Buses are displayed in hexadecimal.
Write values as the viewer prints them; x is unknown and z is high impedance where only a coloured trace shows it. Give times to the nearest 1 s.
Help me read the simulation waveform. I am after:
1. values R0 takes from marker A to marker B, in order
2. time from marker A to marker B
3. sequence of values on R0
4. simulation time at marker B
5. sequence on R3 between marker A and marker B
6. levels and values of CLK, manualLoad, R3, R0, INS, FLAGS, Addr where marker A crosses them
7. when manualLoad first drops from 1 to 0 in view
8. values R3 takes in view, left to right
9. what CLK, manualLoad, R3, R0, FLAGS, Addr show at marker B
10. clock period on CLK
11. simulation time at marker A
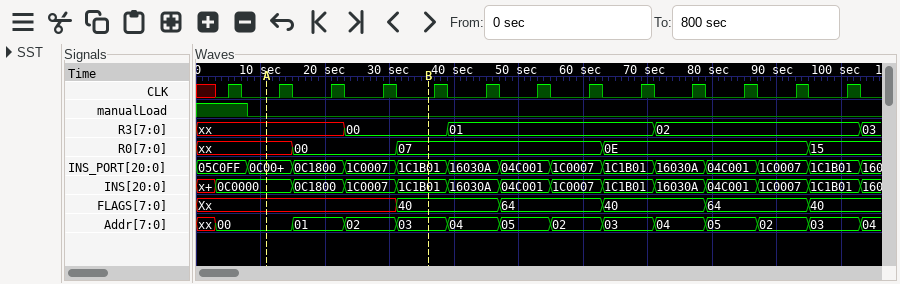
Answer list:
xx, 00, 07
25 s
xx, 00, 07, 0E, 15
36 s
xx, 00
CLK=0, manualLoad=0, R3=xx, R0=xx, INS=0C0000, FLAGS=Xx, Addr=00
8 s
xx, 00, 01, 02, 03
CLK=0, manualLoad=0, R3=00, R0=07, FLAGS=40, Addr=03
8 s
11 s
